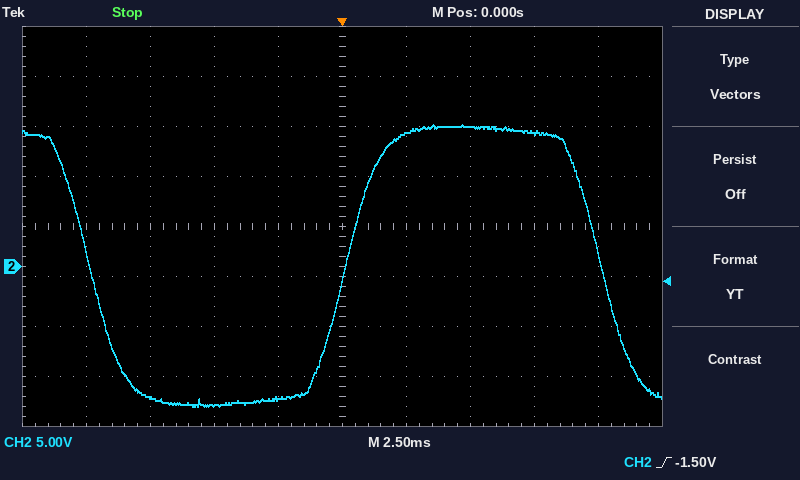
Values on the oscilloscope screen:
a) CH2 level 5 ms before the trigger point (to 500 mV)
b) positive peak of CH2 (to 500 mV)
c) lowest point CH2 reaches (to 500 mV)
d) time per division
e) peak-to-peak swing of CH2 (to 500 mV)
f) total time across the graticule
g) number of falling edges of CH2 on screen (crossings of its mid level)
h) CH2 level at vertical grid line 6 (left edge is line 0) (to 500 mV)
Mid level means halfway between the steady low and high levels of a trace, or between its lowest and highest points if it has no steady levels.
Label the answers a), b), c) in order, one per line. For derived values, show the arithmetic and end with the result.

a) -14.0 V
b) 14.0 V
c) -14.0 V
d) 2.5 ms
e) 14.0 V − (-14.0 V) = 28.0 V
f) 25 ms
g) 2
h) 13.5 V
